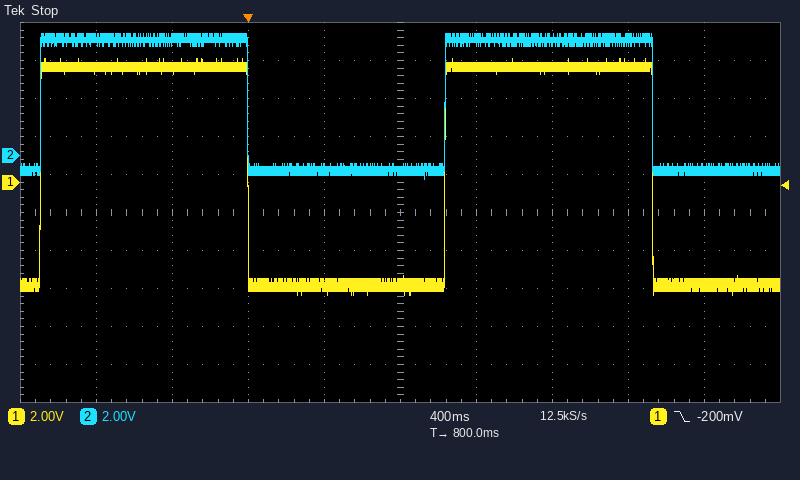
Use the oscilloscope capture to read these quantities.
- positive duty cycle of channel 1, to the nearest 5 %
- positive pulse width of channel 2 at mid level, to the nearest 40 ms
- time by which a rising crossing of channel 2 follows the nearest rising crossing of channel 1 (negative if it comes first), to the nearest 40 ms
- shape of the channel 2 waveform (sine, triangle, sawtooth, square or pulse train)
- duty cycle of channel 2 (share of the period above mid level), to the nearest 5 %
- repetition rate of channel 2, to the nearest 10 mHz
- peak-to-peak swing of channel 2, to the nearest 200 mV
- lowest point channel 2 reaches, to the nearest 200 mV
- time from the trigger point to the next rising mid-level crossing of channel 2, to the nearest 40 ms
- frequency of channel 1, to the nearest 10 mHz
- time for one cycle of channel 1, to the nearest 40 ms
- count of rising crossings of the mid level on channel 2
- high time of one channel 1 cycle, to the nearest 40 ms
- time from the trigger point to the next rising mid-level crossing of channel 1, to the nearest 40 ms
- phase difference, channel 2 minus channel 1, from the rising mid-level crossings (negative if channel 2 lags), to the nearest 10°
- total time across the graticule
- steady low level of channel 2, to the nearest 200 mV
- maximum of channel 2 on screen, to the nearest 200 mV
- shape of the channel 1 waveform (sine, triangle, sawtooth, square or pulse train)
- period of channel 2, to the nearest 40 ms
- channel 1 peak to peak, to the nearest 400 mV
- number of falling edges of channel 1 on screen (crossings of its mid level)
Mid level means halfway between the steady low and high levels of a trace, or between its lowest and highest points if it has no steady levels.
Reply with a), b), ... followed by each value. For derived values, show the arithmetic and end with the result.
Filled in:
a) 1.08 s / 2.12 s ≈ 50.9 %, so 50 % to the nearest 5 %
b) 1.08 s
c) 0 ms
d) square
e) 1.08 s / 2.12 s ≈ 50.9 %, so 50 % to the nearest 5 %
f) 1 / 2.12 s ≈ 472 mHz, so 470 mHz to the nearest 10 mHz
g) 6.4 V − (-1.2 V) = 7.6 V
h) -1.2 V
i) 1.04 s
j) 1 / 2.12 s ≈ 472 mHz, so 470 mHz to the nearest 10 mHz
k) 2.12 s
l) 2
m) 1.08 s
n) 1.04 s
o) −360° × (0 ms) / 2.12 s ≈ 0°
p) 4 s
q) -800 mV
r) 6.4 V
s) square
t) 2.12 s
u) 12.4 V
v) 2
